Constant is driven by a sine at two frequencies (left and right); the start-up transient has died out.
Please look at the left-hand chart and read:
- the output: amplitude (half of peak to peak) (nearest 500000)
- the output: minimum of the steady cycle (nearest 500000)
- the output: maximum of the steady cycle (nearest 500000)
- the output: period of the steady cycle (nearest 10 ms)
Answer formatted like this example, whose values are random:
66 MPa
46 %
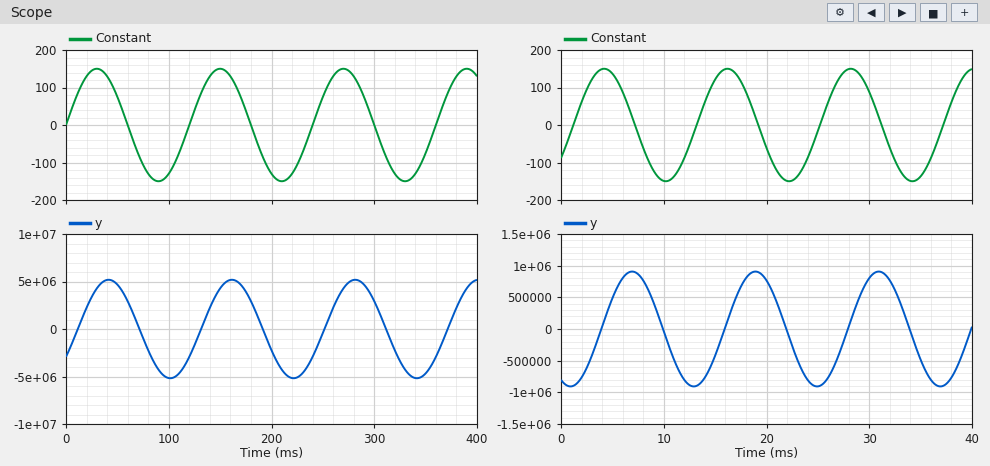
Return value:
5000000
-5000000
5000000
120 ms
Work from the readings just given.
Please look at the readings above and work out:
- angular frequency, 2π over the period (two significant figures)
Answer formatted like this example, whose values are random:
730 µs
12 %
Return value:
0.052 rad/ms
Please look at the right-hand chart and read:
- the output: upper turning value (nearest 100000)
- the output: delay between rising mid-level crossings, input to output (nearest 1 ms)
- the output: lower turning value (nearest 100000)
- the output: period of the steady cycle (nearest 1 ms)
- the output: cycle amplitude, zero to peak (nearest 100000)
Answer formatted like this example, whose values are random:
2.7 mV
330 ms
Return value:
900000
3 ms
-900000
12 ms
900000
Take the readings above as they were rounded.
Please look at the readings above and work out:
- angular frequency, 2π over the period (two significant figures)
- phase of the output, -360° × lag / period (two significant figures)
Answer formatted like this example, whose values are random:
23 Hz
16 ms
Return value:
0.52 rad/ms
-90°
